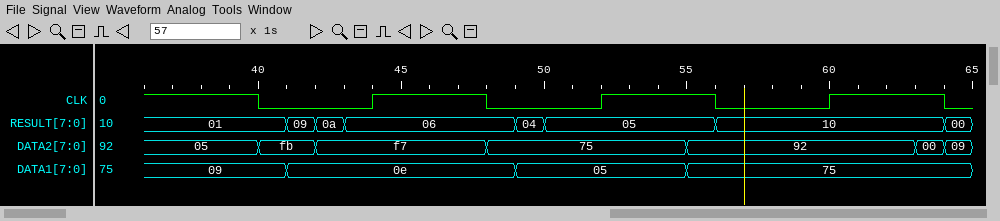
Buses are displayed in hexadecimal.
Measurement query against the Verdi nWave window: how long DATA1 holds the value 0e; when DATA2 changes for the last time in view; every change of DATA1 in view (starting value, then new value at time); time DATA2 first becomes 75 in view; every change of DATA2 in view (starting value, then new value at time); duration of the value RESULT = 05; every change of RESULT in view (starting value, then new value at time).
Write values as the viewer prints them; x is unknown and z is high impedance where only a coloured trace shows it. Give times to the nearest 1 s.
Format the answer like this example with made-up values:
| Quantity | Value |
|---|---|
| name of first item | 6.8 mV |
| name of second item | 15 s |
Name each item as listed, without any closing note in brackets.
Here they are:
| Quantity | Value |
|---|---|
| how long DATA1 holds the value 0e | 8 s |
| when DATA2 changes for the last time in view | 64 s |
| every change of DATA1 in view | 09, 0e at 41 s, 05 at 49 s, 75 at 55 s |
| time DATA2 first becomes 75 in view | 48 s |
| every change of DATA2 in view | 05, fb at 40 s, f7 at 42 s, 75 at 48 s, 92 at 55 s, 00 at 63 s, 09 at 64 s |
| duration of the value RESULT = 05 | 6 s |
| every change of RESULT in view | 01, 09 at 41 s, 0a at 42 s, 06 at 43 s, 04 at 49 s, 05 at 50 s, 10 at 56 s, 00 at 64 s |
